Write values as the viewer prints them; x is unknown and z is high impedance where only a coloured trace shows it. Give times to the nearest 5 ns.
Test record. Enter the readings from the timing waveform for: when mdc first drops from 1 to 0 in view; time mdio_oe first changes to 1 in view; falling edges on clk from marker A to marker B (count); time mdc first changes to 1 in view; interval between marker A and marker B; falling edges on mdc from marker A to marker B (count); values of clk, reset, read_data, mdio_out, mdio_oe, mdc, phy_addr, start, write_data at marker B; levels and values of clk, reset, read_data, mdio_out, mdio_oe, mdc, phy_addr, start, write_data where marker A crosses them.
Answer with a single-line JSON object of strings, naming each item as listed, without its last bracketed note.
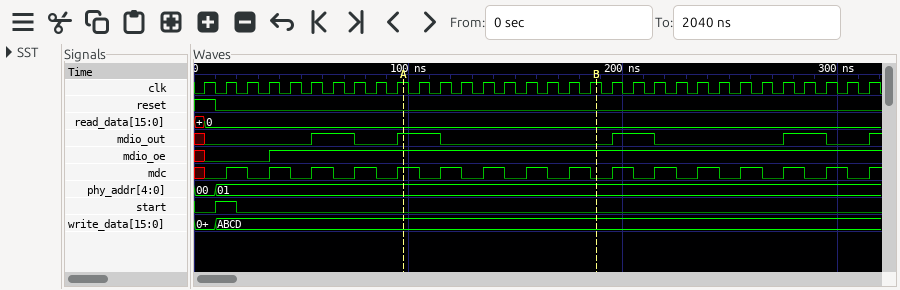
{"when mdc first drops from 1 to 0 in view": "25 ns", "time mdio_oe first changes to 1 in view": "35 ns", "falling edges on clk from marker A to marker B": "9", "time mdc first changes to 1 in view": "15 ns", "interval between marker A and marker B": "90 ns", "falling edges on mdc from marker A to marker B": "5", "values of clk, reset, read_data, mdio_out, mdio_oe, mdc, phy_addr, start, write_data at marker B": "clk=1, reset=0, read_data=0, mdio_out=0, mdio_oe=1, mdc=0, phy_addr=01, start=0, write_data=ABCD", "levels and values of clk, reset, read_data, mdio_out, mdio_oe, mdc, phy_addr, start, write_data where marker A crosses them": "clk=1, reset=0, read_data=0, mdio_out=1, mdio_oe=1, mdc=1, phy_addr=01, start=0, write_data=ABCD"}
